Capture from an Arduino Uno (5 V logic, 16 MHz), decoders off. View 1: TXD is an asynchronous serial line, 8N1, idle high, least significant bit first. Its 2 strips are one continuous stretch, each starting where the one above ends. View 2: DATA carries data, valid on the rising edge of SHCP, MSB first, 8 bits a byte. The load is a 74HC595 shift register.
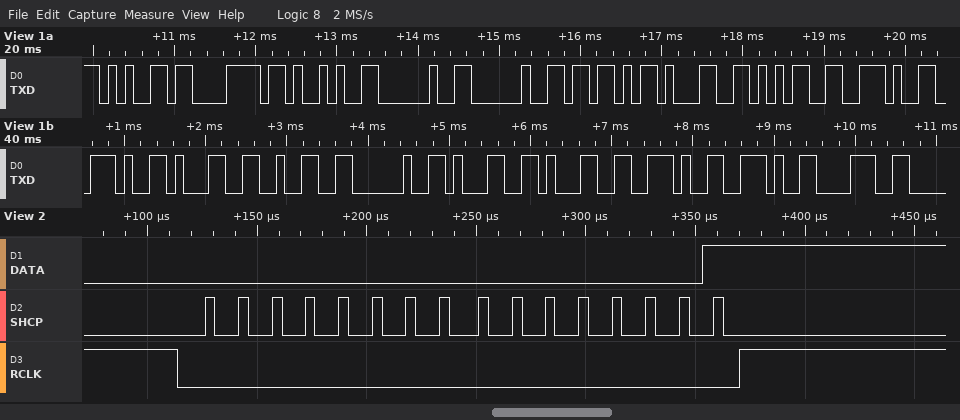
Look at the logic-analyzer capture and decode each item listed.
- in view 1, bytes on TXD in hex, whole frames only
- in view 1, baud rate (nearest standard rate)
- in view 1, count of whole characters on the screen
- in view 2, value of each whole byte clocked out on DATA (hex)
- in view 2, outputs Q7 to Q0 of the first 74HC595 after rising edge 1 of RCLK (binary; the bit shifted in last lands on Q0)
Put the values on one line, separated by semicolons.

0x65 0x78 0x29 0x20 0x20 0x5B 0x31 0x35 0x2E 0x2E 0x31 0x32 0x20 0x31 0x31 0x2E 0x2E 0x38; 9600 baud; 18; 0x00 0x01; 00000001
